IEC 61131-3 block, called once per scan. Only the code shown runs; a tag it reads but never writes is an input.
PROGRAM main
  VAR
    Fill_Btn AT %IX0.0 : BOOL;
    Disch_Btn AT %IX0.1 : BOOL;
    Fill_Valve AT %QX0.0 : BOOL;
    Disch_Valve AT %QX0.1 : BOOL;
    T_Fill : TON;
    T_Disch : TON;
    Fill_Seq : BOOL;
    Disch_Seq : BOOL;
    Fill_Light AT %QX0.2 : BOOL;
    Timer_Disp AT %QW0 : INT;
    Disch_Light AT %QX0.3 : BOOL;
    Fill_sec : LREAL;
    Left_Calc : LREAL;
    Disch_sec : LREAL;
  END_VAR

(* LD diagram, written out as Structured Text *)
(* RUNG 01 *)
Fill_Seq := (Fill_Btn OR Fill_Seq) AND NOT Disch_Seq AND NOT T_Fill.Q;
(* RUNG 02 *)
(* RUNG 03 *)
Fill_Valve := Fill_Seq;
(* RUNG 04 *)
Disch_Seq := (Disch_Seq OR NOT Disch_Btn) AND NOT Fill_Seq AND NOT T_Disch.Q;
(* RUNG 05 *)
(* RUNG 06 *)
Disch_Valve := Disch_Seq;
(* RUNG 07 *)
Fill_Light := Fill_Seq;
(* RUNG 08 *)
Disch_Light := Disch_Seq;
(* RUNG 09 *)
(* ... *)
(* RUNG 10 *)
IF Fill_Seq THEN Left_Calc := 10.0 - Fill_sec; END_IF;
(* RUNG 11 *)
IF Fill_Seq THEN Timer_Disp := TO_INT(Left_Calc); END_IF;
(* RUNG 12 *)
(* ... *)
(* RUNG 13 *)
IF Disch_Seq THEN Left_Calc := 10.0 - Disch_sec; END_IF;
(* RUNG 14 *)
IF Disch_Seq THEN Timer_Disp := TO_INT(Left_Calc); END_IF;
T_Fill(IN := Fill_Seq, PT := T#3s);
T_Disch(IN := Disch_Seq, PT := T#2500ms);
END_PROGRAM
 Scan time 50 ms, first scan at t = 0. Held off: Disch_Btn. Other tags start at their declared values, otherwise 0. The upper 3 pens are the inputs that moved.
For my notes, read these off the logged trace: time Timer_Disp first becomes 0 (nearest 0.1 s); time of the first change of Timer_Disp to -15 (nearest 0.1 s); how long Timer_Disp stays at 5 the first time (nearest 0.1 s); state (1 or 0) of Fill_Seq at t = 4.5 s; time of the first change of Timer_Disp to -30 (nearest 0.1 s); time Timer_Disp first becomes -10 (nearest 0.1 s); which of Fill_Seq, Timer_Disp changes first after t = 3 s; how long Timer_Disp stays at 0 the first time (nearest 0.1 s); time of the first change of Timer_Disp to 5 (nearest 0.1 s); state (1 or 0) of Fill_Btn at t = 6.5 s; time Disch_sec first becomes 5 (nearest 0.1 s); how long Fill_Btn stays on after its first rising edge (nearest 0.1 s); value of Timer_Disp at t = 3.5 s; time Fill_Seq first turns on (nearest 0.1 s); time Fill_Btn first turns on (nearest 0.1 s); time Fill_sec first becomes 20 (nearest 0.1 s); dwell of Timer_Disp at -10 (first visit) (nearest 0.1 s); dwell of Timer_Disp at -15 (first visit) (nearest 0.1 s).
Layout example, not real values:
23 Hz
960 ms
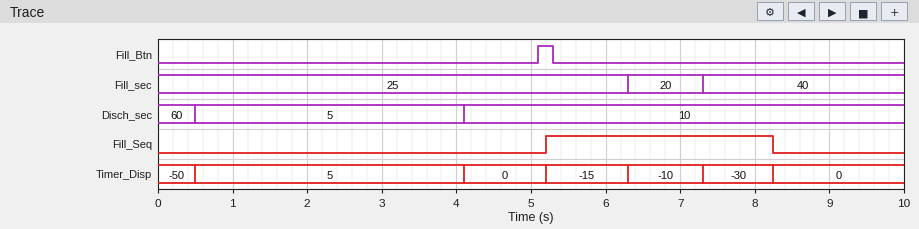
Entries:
4.1 s
5.2 s
3.6 s
0
7.3 s
6.3 s
Timer_Disp
1.1 s
0.5 s
0
0.5 s
0.2 s
5
5.2 s
5.1 s
6.3 s
1.0 s
1.1 s
